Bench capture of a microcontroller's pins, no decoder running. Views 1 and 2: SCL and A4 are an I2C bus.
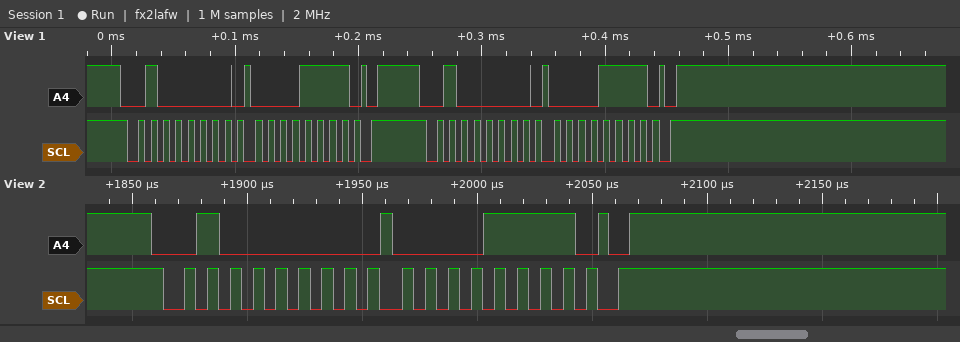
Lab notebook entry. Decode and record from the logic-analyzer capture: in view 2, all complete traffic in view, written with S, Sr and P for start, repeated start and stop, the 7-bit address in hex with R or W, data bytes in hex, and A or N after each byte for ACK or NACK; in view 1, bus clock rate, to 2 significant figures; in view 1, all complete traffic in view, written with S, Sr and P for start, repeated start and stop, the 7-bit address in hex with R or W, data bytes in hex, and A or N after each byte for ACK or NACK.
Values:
S 20W A 0F A P
100 kHz
S 20W A 0F A P S 20W A 0F A P
